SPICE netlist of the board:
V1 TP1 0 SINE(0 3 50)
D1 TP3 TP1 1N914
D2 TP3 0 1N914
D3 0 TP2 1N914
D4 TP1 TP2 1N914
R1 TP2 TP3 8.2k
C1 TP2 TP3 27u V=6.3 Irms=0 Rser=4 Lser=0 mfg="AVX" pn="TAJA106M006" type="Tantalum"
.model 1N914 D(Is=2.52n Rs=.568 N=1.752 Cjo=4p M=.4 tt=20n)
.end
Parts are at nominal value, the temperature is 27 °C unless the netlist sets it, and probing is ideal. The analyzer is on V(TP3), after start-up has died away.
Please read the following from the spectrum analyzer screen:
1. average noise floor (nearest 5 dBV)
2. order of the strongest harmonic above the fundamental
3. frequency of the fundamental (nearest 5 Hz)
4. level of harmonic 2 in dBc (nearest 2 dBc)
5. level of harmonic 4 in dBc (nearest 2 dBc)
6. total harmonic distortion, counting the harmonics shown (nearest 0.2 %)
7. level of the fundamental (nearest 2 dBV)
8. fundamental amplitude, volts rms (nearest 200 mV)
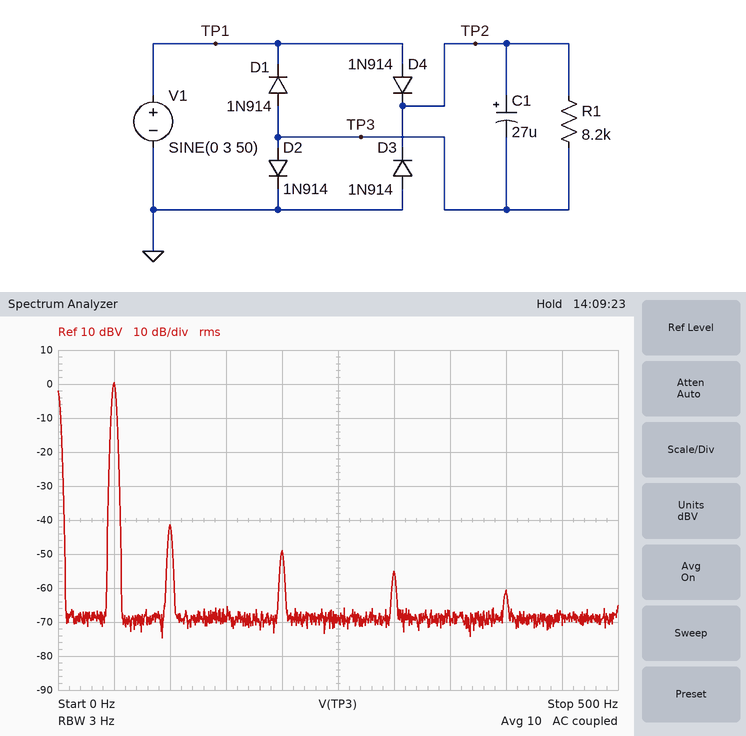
-70 dBV
2
50 Hz
-42 dBc
-50 dBc
0.8 %
0 dBV
1.0 V
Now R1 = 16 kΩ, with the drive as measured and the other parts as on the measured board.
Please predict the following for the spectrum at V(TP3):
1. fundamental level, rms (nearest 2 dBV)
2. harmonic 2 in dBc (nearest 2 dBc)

0 dBV
-48 dBc
